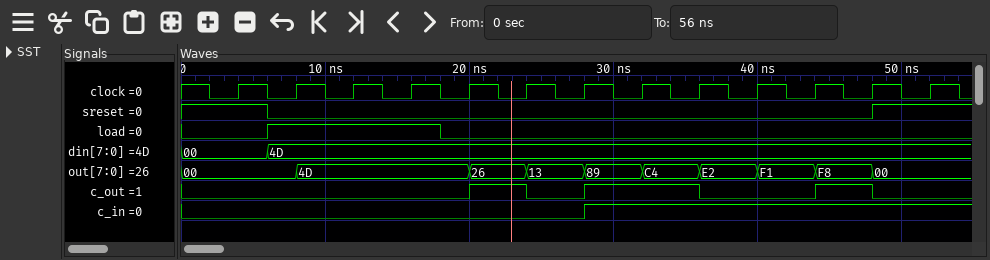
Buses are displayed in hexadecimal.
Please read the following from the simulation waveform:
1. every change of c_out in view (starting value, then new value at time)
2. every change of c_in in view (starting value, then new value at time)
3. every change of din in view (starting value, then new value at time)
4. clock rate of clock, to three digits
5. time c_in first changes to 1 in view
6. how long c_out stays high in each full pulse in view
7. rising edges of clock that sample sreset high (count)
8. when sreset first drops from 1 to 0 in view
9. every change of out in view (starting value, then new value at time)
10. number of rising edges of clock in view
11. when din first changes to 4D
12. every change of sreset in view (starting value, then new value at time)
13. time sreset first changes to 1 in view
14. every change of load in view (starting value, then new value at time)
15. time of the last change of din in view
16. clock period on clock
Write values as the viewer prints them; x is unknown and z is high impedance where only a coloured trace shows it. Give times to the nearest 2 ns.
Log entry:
0, 1 at 20 ns, 0 at 24 ns, 1 at 28 ns, 0 at 36 ns, 1 at 44 ns, 0 at 48 ns
0, 1 at 28 ns
00, 4D at 6 ns
250 MHz
28 ns
4 ns, 8 ns, 4 ns
2
6 ns
00, 4D at 8 ns, 26 at 20 ns, 13 at 24 ns, 89 at 28 ns, C4 at 32 ns, E2 at 36 ns, F1 at 40 ns, F8 at 44 ns, 00 at 48 ns
13
6 ns
1, 0 at 6 ns, 1 at 48 ns
48 ns
0, 1 at 6 ns, 0 at 18 ns
6 ns
4 ns
